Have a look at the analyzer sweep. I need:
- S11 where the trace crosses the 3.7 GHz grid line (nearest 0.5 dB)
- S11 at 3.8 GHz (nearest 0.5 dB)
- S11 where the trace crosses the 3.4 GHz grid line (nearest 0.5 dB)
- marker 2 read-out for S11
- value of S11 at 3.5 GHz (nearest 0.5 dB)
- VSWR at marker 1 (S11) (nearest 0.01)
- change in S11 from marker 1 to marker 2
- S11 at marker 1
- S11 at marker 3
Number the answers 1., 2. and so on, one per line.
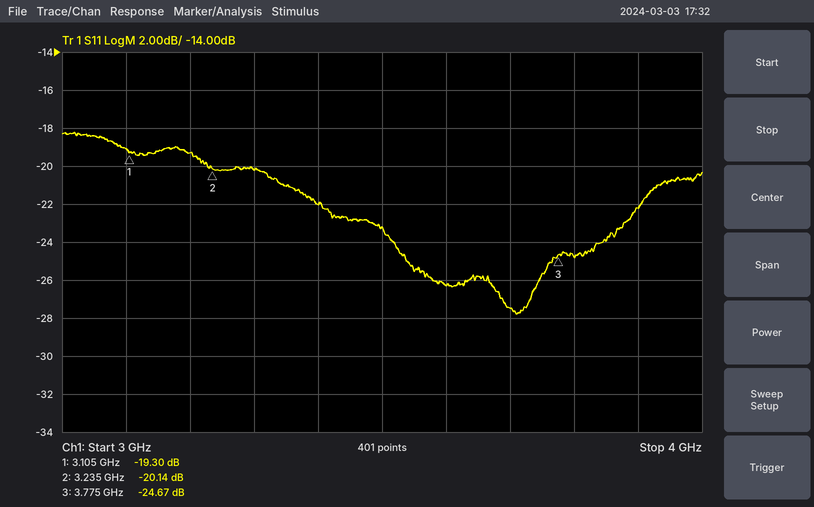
1. -27.5 dB
2. -25.0 dB
3. -22.0 dB
4. -20.14 dB
5. -23.0 dB
6. 1.24
7. -0.84 dB
8. -19.30 dB
9. -24.67 dB
